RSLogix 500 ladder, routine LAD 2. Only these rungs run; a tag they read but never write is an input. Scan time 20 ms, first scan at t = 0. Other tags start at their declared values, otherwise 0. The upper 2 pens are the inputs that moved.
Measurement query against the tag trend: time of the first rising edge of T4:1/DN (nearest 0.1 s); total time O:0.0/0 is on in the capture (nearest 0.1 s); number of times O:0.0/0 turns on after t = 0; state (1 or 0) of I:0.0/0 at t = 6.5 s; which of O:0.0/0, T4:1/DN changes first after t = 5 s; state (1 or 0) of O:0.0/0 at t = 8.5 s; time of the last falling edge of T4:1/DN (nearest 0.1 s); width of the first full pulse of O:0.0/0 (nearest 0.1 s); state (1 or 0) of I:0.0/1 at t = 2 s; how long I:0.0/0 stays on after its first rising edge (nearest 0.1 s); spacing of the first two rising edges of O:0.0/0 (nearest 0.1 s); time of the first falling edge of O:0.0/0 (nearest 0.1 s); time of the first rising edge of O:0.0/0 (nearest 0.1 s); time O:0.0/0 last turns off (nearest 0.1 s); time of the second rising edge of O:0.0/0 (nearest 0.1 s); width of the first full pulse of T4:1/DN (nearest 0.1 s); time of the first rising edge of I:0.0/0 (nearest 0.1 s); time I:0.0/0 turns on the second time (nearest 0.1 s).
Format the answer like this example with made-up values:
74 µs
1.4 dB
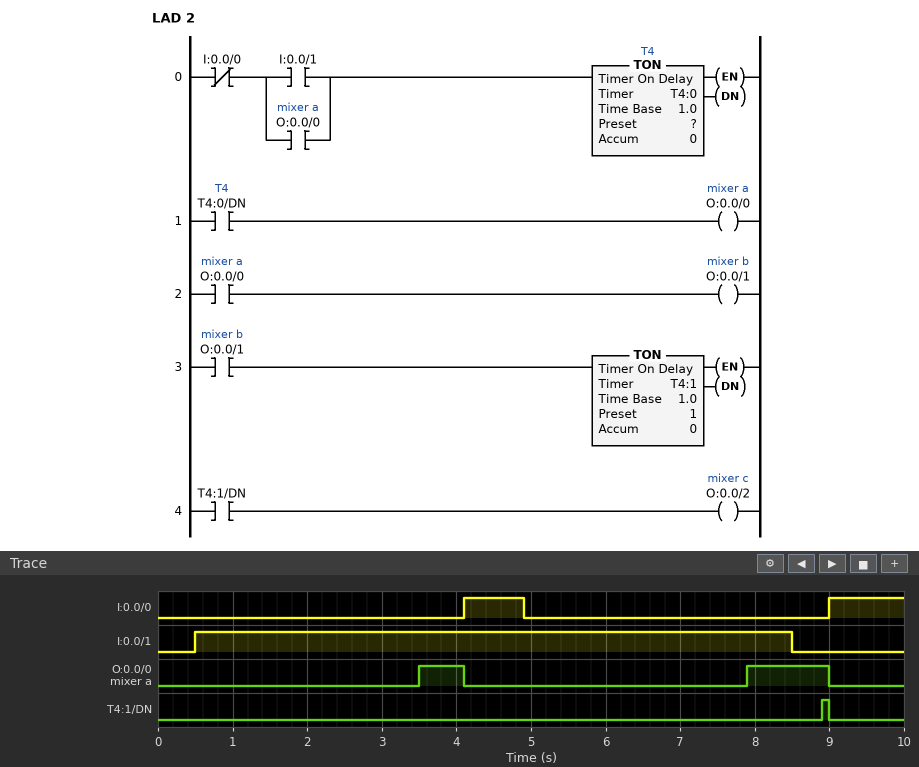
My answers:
8.9 s
1.7 s
2
0
O:0.0/0
1
9.0 s
0.6 s
1
0.8 s
4.4 s
4.1 s
3.5 s
9.0 s
7.9 s
0.1 s
4.1 s
9.0 s
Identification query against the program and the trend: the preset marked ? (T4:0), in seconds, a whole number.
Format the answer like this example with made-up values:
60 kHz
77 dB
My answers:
3 s
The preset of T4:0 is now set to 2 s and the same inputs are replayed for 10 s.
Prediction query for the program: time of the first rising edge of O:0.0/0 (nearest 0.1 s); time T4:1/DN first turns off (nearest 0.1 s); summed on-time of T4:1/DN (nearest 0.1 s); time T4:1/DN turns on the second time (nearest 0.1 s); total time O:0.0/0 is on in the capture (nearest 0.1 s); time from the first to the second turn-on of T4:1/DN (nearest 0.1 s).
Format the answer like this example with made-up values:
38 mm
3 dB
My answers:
2.5 s
4.1 s
1.7 s
7.9 s
3.7 s
4.4 s
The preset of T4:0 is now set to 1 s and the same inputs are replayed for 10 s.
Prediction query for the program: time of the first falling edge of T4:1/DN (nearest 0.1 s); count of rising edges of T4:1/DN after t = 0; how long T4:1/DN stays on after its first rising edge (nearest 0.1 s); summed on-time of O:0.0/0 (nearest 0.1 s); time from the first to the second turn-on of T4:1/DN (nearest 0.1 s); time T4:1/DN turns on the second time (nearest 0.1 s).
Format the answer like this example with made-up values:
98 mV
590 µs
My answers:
4.1 s
2
1.6 s
5.7 s
4.4 s
6.9 s
